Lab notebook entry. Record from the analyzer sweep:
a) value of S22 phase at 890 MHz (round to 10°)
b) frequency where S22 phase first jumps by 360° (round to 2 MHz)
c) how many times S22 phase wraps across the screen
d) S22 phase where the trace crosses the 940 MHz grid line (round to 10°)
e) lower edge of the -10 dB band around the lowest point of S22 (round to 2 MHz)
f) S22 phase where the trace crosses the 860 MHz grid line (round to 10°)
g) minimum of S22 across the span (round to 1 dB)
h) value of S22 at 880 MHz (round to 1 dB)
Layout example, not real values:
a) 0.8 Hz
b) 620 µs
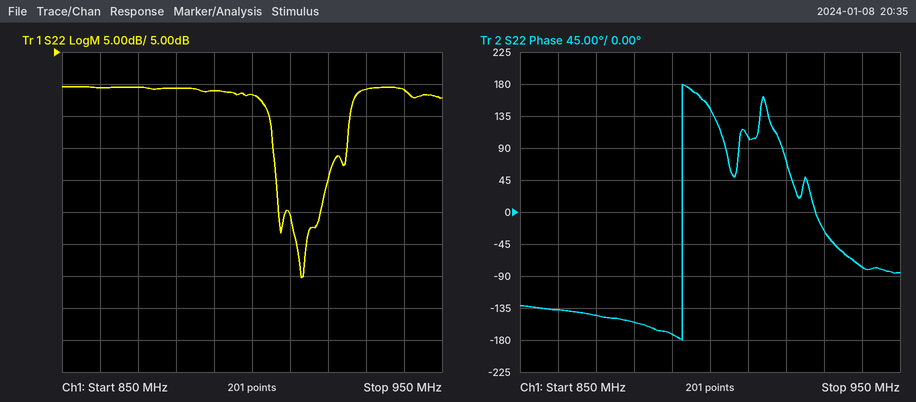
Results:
a) -170°
b) 892 MHz
c) 1
d) -80°
e) 906 MHz
f) -140°
g) -30 dB
h) -1 dB
